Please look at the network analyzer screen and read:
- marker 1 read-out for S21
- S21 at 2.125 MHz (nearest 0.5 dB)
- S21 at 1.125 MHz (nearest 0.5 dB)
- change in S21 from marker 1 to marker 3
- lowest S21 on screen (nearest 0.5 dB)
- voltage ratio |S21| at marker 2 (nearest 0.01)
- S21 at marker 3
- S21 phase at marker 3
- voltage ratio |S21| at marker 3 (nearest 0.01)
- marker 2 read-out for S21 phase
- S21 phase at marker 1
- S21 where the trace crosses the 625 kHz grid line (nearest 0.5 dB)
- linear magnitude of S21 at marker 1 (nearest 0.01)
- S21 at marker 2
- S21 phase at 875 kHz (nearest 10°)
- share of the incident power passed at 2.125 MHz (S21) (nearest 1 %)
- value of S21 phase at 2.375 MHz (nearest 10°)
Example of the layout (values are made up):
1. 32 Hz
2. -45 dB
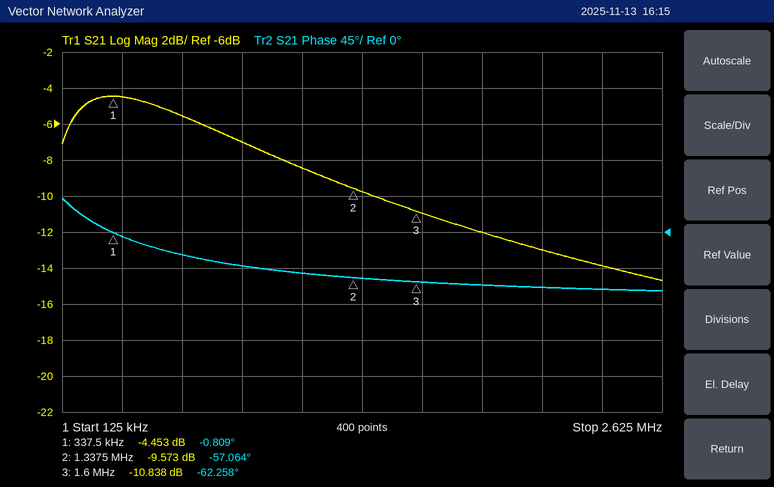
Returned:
1. -4.453 dB
2. -13.0 dB
3. -8.5 dB
4. -6.385 dB
5. -14.5 dB
6. 0.33
7. -10.838 dB
8. -62.258°
9. 0.29
10. -57.064°
11. -0.809°
12. -5.5 dB
13. 0.60
14. -9.573 dB
15. -40°
16. 5 %
17. -70°
